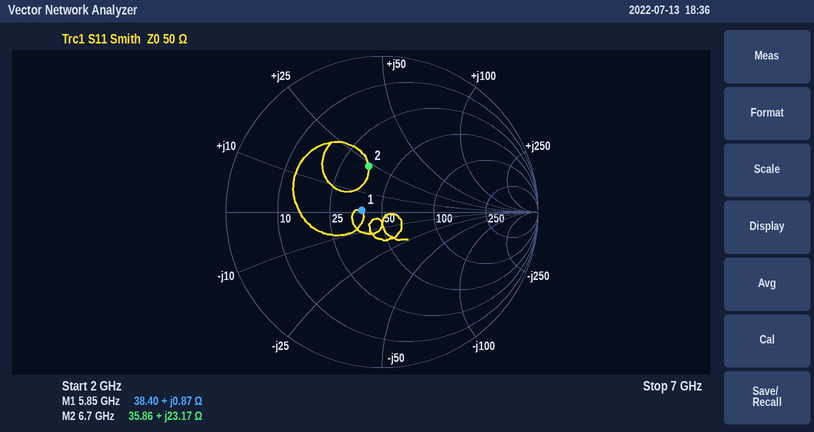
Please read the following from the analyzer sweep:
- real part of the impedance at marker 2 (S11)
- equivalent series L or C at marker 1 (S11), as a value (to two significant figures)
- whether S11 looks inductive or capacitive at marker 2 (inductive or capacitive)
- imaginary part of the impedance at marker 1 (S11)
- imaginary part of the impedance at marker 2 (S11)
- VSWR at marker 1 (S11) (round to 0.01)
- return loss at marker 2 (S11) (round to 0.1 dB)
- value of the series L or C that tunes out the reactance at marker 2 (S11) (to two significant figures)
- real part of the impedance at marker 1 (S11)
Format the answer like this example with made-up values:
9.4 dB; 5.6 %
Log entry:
35.86 Ω; 24 pH; inductive; +0.87 Ω; +23.17 Ω; 1.30; 10.3 dB; 1.0 pF; 38.40 Ω
